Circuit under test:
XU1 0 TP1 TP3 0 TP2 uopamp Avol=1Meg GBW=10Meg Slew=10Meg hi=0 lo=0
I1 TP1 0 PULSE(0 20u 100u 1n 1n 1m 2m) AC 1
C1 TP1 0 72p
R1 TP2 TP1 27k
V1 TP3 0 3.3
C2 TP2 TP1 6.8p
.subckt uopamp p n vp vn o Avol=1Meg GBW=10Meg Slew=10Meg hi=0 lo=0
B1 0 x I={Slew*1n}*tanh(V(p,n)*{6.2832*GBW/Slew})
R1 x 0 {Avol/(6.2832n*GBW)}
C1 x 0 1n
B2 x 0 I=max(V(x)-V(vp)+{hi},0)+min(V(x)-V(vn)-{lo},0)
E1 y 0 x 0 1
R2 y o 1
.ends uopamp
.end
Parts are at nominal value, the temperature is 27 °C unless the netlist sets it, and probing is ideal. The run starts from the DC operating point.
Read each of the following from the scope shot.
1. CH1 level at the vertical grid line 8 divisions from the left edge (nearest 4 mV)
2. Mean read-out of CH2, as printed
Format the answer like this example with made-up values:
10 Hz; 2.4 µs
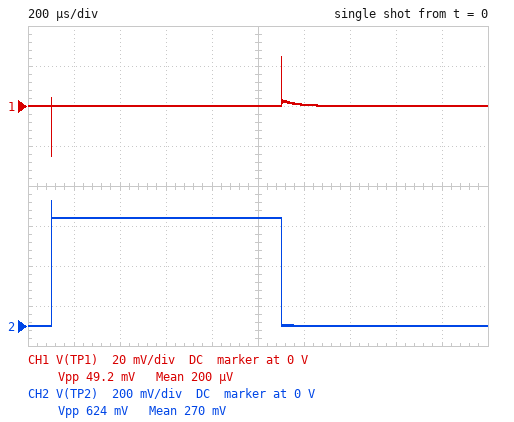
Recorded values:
0 V; 270 mV
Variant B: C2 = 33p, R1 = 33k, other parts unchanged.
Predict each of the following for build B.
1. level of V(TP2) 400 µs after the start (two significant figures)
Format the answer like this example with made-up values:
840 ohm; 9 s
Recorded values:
660 mV
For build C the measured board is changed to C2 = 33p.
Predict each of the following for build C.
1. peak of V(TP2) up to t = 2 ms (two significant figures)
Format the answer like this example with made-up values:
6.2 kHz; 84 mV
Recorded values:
540 mV
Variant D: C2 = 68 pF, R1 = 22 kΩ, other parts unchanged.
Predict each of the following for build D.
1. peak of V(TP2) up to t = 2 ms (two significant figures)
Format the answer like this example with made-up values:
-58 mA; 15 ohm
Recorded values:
440 mV
